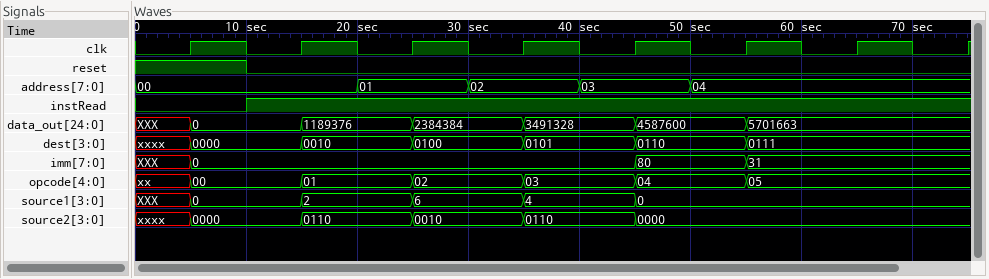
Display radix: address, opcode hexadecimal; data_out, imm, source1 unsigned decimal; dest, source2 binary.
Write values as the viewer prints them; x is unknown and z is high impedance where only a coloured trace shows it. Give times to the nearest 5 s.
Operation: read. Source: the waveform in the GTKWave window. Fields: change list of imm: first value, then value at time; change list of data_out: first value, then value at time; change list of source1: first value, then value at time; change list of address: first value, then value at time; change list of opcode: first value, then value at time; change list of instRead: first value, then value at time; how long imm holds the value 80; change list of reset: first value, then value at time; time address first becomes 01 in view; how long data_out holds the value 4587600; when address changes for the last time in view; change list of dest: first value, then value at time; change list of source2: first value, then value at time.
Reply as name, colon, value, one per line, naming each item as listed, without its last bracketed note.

change list of imm: first value, then value at time: XXX, 0 at 5 s, 80 at 45 s, 31 at 55 s
change list of data_out: first value, then value at time: XXX, 0 at 5 s, 1189376 at 15 s, 2384384 at 25 s, 3491328 at 35 s, 4587600 at 45 s, 5701663 at 55 s
change list of source1: first value, then value at time: XXX, 0 at 5 s, 2 at 15 s, 6 at 25 s, 4 at 35 s, 0 at 45 s
change list of address: first value, then value at time: 00, 01 at 20 s, 02 at 30 s, 03 at 40 s, 04 at 50 s
change list of opcode: first value, then value at time: xx, 00 at 5 s, 01 at 15 s, 02 at 25 s, 03 at 35 s, 04 at 45 s, 05 at 55 s
change list of instRead: first value, then value at time: 0, 1 at 10 s
how long imm holds the value 80: 10 s
change list of reset: first value, then value at time: 1, 0 at 10 s
time address first becomes 01 in view: 20 s
how long data_out holds the value 4587600: 10 s
when address changes for the last time in view: 50 s
change list of dest: first value, then value at time: xxxx, 0000 at 5 s, 0010 at 15 s, 0100 at 25 s, 0101 at 35 s, 0110 at 45 s, 0111 at 55 s
change list of source2: first value, then value at time: xxxx, 0000 at 5 s, 0110 at 15 s, 0010 at 25 s, 0110 at 35 s, 0000 at 45 s
